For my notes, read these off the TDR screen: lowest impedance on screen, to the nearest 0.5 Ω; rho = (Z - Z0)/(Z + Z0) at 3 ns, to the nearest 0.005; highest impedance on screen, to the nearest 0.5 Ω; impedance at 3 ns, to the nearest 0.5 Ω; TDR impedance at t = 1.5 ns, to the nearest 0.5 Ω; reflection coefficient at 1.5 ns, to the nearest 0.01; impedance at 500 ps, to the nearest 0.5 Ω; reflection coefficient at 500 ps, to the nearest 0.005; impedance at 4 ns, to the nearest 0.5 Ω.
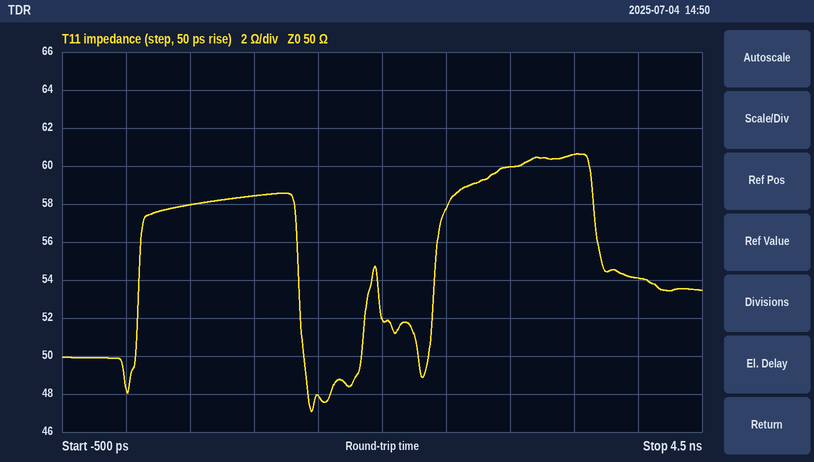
47.0 Ω
+0.090
60.5 Ω
60.0 Ω
48.0 Ω
-0.02
58.0 Ω
+0.075
54.0 Ω
